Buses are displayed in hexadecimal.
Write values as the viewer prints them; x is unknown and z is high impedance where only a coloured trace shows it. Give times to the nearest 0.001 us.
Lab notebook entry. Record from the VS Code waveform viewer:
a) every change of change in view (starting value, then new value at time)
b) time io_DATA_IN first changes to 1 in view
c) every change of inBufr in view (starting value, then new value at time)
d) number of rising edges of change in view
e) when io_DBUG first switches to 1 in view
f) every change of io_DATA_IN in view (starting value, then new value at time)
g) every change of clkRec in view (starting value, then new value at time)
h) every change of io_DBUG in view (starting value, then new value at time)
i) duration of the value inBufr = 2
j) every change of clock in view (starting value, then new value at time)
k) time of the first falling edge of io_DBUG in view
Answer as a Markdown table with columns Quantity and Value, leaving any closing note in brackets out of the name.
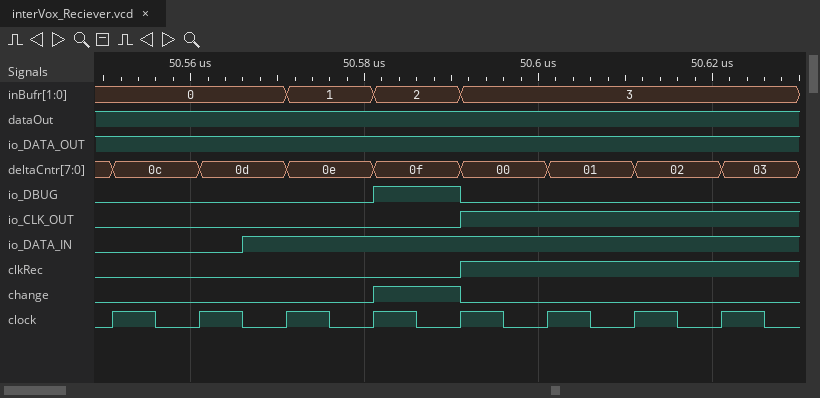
| Quantity | Value |
|---|---|
| every change of change in view | 0, 1 at 50.581 us, 0 at 50.591 us |
| time io_DATA_IN first changes to 1 in view | 50.566 us |
| every change of inBufr in view | 0, 1 at 50.571 us, 2 at 50.581 us, 3 at 50.591 us |
| number of rising edges of change in view | 1 |
| when io_DBUG first switches to 1 in view | 50.581 us |
| every change of io_DATA_IN in view | 0, 1 at 50.566 us |
| every change of clkRec in view | 0, 1 at 50.591 us |
| every change of io_DBUG in view | 0, 1 at 50.581 us, 0 at 50.591 us |
| duration of the value inBufr = 2 | 0.01 us |
| every change of clock in view | 0, 1 at 50.551 us, 0 at 50.556 us, 1 at 50.561 us, 0 at 50.566 us, 1 at 50.571 us, 0 at 50.576 us, 1 at 50.581 us, 0 at 50.586 us, 1 at 50.591 us, 0 at 50.596 us, 1 at 50.601 us, 0 at 50.606 us, 1 at 50.611 us, 0 at 50.616 us, 1 at 50.621 us, 0 at 50.626 us |
| time of the first falling edge of io_DBUG in view | 50.591 us |
